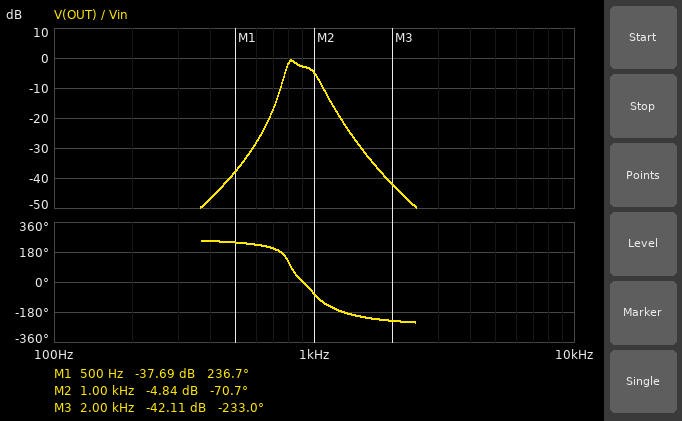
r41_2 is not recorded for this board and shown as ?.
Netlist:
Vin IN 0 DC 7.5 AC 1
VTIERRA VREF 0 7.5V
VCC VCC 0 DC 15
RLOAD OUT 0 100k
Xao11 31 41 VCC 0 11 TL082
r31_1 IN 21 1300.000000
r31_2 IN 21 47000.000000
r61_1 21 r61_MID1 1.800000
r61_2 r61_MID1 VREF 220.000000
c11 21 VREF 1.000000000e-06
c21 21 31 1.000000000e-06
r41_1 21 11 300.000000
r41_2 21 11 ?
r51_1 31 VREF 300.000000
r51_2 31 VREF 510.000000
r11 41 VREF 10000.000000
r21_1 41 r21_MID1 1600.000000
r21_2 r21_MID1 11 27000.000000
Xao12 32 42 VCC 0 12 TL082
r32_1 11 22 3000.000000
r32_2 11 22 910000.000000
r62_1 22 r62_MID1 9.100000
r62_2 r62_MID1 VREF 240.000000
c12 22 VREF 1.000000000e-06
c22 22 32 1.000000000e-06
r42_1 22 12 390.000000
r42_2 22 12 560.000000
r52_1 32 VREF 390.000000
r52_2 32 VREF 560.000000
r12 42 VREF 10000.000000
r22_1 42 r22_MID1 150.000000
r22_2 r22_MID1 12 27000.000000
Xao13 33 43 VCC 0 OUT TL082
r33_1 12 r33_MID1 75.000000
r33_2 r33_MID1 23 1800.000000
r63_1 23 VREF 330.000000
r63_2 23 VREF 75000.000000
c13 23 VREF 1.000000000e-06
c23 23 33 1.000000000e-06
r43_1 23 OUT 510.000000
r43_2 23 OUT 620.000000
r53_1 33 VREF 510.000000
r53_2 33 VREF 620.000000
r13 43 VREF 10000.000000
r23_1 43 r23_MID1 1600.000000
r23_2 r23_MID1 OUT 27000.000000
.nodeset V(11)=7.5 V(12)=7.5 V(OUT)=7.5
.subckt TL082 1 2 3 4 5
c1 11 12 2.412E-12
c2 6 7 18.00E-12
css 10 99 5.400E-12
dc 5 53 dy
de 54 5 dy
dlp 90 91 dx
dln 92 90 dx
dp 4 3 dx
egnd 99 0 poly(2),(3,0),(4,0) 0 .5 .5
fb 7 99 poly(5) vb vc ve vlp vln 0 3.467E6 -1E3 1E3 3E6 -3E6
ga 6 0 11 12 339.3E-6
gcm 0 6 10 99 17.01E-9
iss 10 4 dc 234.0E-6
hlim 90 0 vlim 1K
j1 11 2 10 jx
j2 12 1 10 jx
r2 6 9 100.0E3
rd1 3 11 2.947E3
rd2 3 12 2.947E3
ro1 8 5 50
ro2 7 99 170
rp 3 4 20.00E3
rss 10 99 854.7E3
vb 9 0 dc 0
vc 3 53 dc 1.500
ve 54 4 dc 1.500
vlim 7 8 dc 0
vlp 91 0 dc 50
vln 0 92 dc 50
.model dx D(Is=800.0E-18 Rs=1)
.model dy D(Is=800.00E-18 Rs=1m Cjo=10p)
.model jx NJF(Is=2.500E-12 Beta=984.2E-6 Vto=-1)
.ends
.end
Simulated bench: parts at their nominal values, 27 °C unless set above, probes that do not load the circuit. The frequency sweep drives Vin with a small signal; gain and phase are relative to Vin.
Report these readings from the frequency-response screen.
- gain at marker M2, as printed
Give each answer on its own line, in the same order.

-4.84 dB
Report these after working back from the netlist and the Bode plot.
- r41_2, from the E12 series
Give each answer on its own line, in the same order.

1.5 kΩ
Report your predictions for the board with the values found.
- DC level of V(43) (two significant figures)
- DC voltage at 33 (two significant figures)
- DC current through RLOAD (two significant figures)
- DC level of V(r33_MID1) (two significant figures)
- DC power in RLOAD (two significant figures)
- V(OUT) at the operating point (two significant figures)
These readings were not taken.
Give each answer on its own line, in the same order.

7.5 V
7.5 V
75 µA
7.5 V
560 µW
7.5 V
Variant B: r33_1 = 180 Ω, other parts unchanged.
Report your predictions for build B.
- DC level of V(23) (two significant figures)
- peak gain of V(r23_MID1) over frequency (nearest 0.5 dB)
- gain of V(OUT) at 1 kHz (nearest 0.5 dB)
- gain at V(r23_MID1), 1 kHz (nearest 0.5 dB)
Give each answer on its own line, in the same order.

7.5 V
-11.5 dB
-5.5 dB
-16.0 dB
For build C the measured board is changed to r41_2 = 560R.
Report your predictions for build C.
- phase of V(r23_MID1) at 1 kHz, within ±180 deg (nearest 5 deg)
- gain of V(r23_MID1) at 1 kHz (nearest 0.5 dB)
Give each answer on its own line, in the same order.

-25 deg
-10.5 dB
